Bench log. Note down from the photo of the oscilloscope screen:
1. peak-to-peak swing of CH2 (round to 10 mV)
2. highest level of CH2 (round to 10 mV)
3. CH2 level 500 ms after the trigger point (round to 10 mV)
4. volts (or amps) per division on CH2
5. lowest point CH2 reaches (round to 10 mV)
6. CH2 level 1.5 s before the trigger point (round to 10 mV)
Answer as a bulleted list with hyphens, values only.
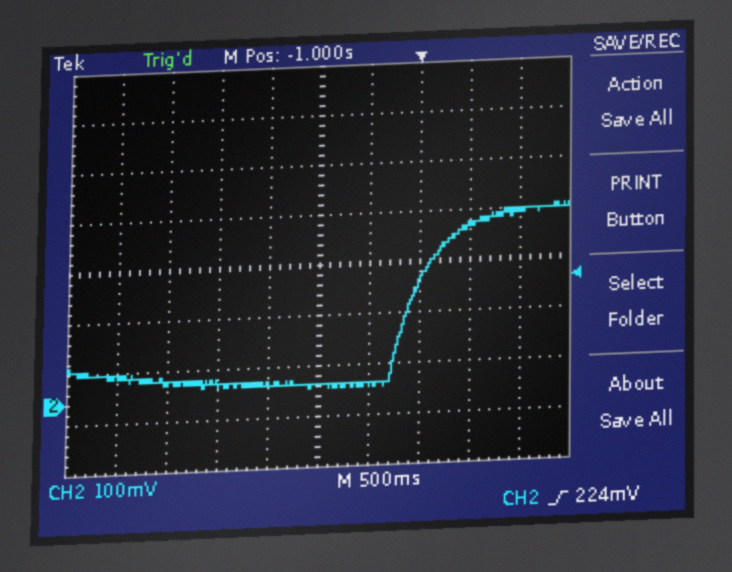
- 350 mV
- 370 mV
- 330 mV
- 100 mV
- 20 mV
- 30 mV
